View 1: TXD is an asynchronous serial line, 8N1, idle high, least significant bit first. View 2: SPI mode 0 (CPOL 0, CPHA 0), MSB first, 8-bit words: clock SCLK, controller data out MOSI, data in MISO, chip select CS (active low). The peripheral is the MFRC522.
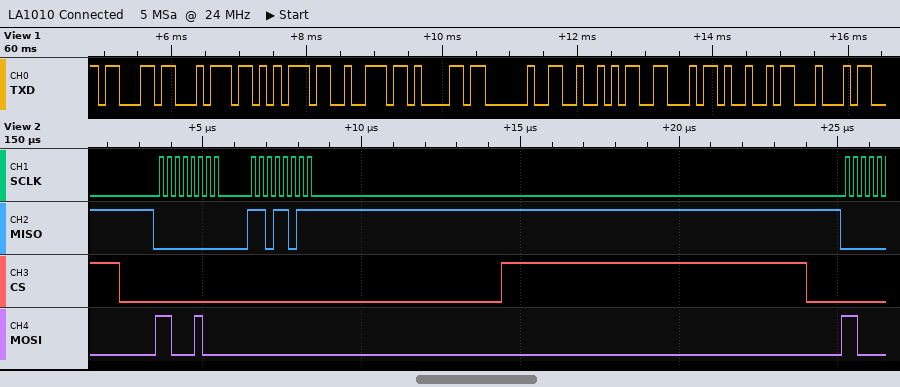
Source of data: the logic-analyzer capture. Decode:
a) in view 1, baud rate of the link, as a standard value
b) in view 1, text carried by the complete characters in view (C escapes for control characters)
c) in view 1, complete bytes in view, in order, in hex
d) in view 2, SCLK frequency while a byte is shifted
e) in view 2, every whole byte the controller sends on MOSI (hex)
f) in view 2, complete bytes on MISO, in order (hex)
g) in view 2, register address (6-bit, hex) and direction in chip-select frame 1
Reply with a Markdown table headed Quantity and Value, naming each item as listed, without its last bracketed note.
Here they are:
| Quantity | Value |
|---|---|
| in view 1, baud rate of the link, as a standard value | 9600 baud |
| in view 1, text carried by the complete characters in view | "ctura RFID" |
| in view 1, complete bytes in view, in order, in hex | 63 74 75 72 61 20 52 46 49 44 |
| in view 2, SCLK frequency while a byte is shifted | 4 MHz |
| in view 2, every whole byte the controller sends on MOSI | 0xC4 0x00 |
| in view 2, complete bytes on MISO, in order | 0x00 0xDB |
| in view 2, register address (6-bit, hex) and direction in chip-select frame 1 | 0x22 read |
